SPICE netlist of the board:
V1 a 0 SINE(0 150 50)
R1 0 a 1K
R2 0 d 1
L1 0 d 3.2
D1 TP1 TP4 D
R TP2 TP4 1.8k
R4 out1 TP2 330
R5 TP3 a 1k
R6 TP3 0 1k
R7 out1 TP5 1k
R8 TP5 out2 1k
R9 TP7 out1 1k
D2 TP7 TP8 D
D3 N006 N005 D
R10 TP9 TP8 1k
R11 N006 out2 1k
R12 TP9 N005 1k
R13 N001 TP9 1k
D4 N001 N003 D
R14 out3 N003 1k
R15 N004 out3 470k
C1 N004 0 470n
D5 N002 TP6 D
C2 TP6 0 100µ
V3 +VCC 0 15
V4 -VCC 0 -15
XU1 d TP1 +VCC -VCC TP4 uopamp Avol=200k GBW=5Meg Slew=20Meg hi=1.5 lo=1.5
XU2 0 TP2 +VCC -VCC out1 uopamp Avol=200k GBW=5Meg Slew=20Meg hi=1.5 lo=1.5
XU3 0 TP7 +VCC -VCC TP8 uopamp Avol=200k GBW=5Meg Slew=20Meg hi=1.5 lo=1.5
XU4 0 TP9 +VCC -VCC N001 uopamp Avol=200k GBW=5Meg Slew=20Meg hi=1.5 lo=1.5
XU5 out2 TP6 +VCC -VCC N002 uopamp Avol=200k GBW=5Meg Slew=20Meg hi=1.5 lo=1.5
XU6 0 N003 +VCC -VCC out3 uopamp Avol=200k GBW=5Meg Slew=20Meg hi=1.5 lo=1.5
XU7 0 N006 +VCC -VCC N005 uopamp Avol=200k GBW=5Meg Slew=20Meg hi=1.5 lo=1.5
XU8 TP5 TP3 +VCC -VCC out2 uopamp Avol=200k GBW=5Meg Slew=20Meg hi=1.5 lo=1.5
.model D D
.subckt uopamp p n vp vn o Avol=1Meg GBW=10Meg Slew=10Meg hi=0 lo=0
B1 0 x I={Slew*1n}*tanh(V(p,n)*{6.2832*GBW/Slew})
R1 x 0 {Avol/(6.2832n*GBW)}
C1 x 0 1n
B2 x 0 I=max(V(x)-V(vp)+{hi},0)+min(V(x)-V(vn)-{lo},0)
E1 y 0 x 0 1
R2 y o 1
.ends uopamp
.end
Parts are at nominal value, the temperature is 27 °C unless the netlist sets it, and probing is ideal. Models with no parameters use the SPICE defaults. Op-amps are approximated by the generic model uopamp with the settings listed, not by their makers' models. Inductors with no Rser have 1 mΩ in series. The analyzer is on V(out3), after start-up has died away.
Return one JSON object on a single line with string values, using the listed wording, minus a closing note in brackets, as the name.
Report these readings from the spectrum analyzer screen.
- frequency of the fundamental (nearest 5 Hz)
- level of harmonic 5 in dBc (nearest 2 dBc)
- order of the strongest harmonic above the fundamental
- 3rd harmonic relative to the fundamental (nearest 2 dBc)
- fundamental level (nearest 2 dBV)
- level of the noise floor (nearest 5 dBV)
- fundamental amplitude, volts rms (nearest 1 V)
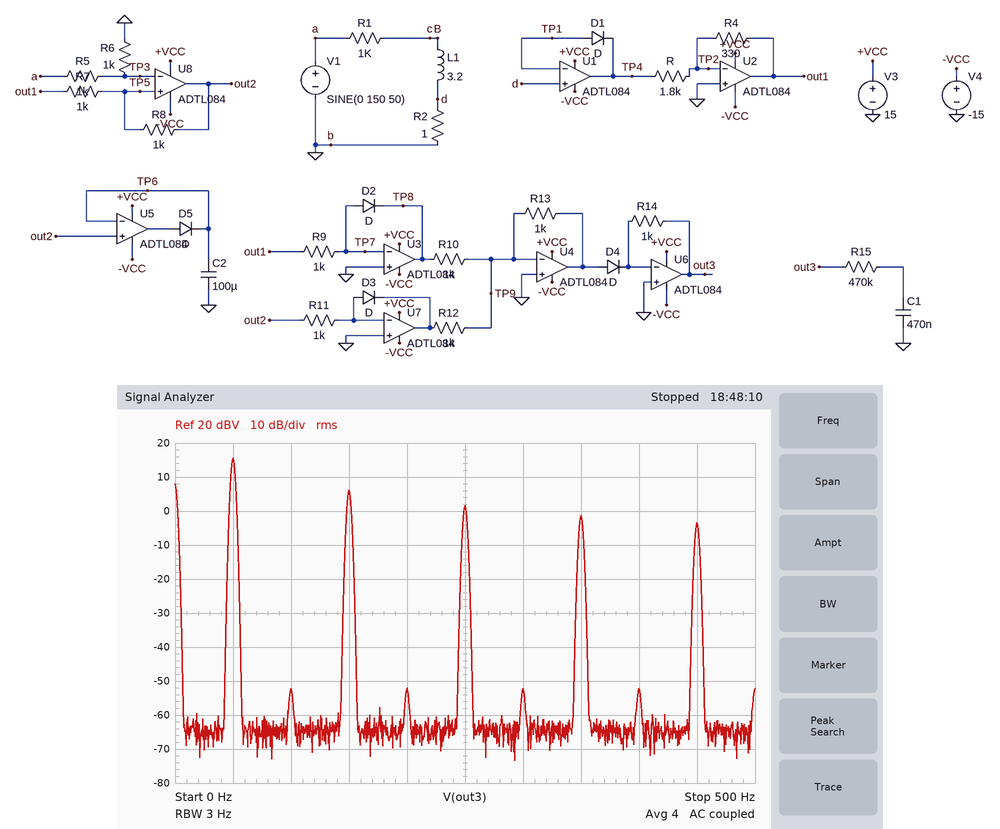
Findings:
{"frequency of the fundamental": "50 Hz", "level of harmonic 5 in dBc": "-14 dBc", "order of the strongest harmonic above the fundamental": "3", "3rd harmonic relative to the fundamental": "-10 dBc", "fundamental level": "16 dBV", "level of the noise floor": "-65 dBV", "fundamental amplitude, volts rms": "6 V"}
